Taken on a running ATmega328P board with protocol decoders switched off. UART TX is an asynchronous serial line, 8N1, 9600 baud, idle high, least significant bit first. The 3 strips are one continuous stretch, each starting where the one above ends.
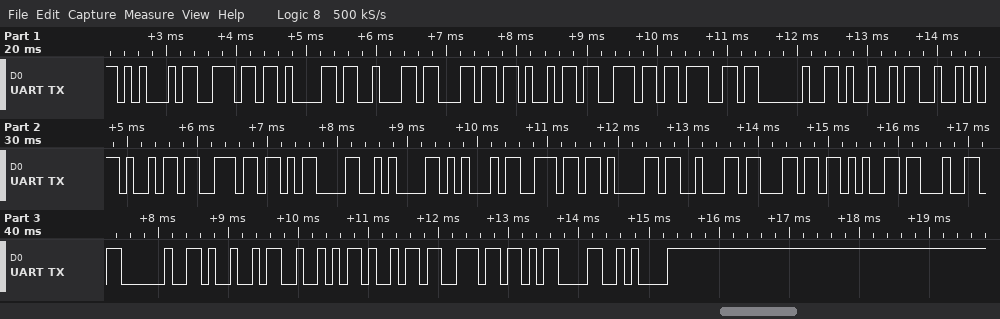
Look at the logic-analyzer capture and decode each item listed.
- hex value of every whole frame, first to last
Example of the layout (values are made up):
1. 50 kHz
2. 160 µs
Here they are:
1. 45 6E 61 62 6C 69 6E 67 20 49 52 69 6E 0D 0A 45 6E 61 62 6C 65 64 20 49 52 69 6E 0D 0A
